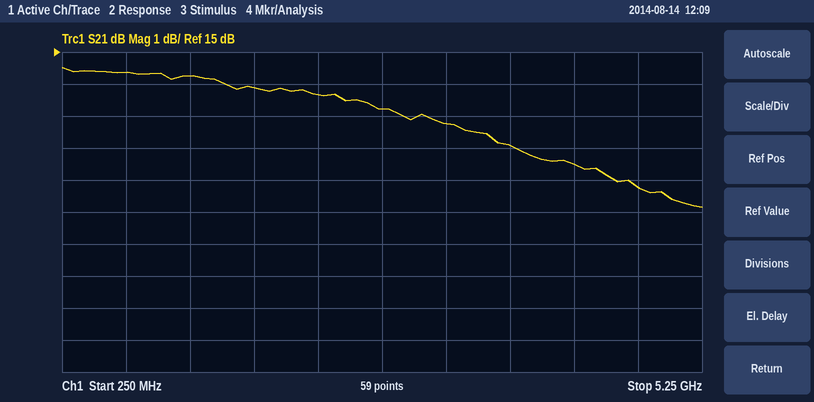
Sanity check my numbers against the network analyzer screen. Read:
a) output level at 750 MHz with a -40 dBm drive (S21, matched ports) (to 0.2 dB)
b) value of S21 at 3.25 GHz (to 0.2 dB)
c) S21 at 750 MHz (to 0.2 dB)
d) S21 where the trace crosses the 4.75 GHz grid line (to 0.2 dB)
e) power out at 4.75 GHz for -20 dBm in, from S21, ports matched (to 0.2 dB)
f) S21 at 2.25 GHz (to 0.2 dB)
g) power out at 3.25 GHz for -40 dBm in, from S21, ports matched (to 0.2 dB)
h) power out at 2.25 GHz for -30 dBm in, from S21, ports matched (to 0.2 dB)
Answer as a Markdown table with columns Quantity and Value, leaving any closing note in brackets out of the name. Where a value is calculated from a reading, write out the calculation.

| Quantity | Value |
|---|---|
| output level at 750 MHz with a -40 dBm drive (S21, matched ports) | -40 dBm + (14.4 dB) = -25.6 dBm |
| value of S21 at 3.25 GHz | 12.8 dB |
| S21 at 750 MHz | 14.4 dB |
| S21 where the trace crosses the 4.75 GHz grid line | 10.8 dB |
| power out at 4.75 GHz for -20 dBm in, from S21, ports matched | -20 dBm + (10.8 dB) = -9.2 dBm |
| S21 at 2.25 GHz | 13.6 dB |
| power out at 3.25 GHz for -40 dBm in, from S21, ports matched | -40 dBm + (12.8 dB) = -27.2 dBm |
| power out at 2.25 GHz for -30 dBm in, from S21, ports matched | -30 dBm + (13.6 dB) = -16.4 dBm |
